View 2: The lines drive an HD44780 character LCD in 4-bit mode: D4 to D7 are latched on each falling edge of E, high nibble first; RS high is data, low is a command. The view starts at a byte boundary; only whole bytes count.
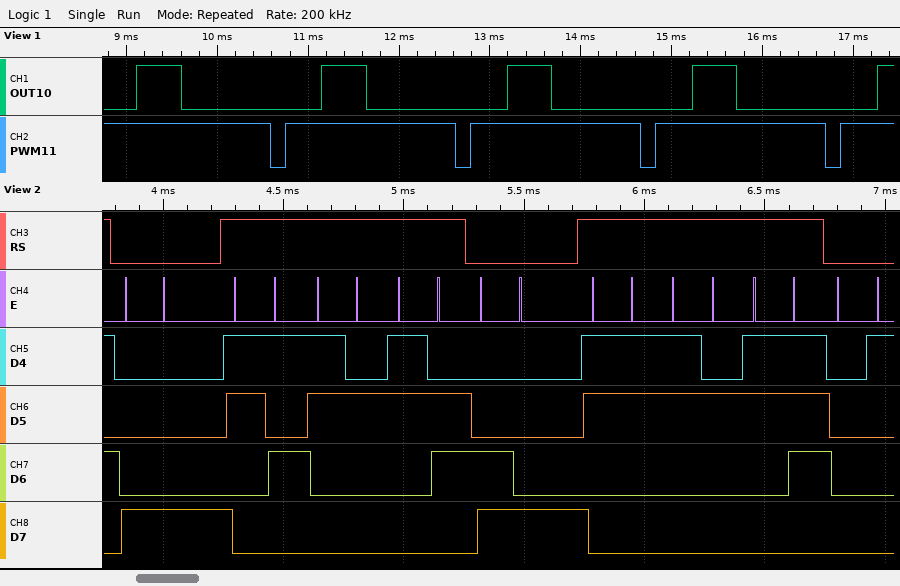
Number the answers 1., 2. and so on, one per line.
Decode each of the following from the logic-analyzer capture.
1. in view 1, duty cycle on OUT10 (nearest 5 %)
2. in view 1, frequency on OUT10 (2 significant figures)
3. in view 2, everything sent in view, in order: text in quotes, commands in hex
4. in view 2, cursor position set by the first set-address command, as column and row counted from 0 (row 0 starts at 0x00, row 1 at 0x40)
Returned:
1. 25 %
2. 490 Hz
3. 0x88 "526" 0xC8 "327" 0x01
4. column 8, row 0
